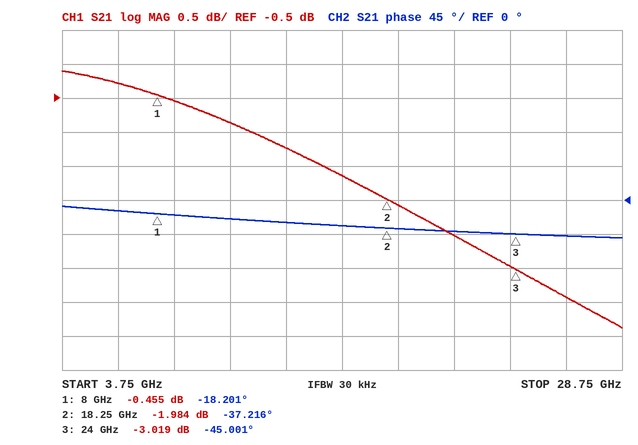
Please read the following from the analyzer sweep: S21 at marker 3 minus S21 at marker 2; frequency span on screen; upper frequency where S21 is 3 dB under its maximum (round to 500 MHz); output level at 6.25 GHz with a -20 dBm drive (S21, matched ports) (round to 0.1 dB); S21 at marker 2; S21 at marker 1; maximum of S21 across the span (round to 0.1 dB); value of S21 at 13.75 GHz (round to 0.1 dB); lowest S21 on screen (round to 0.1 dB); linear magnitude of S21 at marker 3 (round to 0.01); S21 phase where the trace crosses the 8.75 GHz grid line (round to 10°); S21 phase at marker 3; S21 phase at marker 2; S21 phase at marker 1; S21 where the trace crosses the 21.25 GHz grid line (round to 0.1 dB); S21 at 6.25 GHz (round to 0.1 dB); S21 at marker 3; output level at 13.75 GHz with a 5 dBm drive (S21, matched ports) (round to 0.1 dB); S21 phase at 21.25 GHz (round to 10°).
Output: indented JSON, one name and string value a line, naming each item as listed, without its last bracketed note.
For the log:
{
  "S21 at marker 3 minus S21 at marker 2": "-1.035 dB",
  "frequency span on screen": "25 GHz",
  "upper frequency where S21 is 3 dB under its maximum": "24.5 GHz",
  "output level at 6.25 GHz with a -20 dBm drive (S21, matched ports)": "-20.3 dBm",
  "S21 at marker 2": "-1.984 dB",
  "S21 at marker 1": "-0.455 dB",
  "maximum of S21 across the span": "-0.1 dB",
  "value of S21 at 13.75 GHz": "-1.2 dB",
  "lowest S21 on screen": "-3.9 dB",
  "linear magnitude of S21 at marker 3": "0.71",
  "S21 phase where the trace crosses the 8.75 GHz grid line": "-20°",
  "S21 phase at marker 3": "-45.001°",
  "S21 phase at marker 2": "-37.216°",
  "S21 phase at marker 1": "-18.201°",
  "S21 where the trace crosses the 21.25 GHz grid line": "-2.5 dB",
  "S21 at 6.25 GHz": "-0.3 dB",
  "S21 at marker 3": "-3.019 dB",
  "output level at 13.75 GHz with a 5 dBm drive (S21, matched ports)": "3.8 dBm",
  "S21 phase at 21.25 GHz": "-40°"
}
